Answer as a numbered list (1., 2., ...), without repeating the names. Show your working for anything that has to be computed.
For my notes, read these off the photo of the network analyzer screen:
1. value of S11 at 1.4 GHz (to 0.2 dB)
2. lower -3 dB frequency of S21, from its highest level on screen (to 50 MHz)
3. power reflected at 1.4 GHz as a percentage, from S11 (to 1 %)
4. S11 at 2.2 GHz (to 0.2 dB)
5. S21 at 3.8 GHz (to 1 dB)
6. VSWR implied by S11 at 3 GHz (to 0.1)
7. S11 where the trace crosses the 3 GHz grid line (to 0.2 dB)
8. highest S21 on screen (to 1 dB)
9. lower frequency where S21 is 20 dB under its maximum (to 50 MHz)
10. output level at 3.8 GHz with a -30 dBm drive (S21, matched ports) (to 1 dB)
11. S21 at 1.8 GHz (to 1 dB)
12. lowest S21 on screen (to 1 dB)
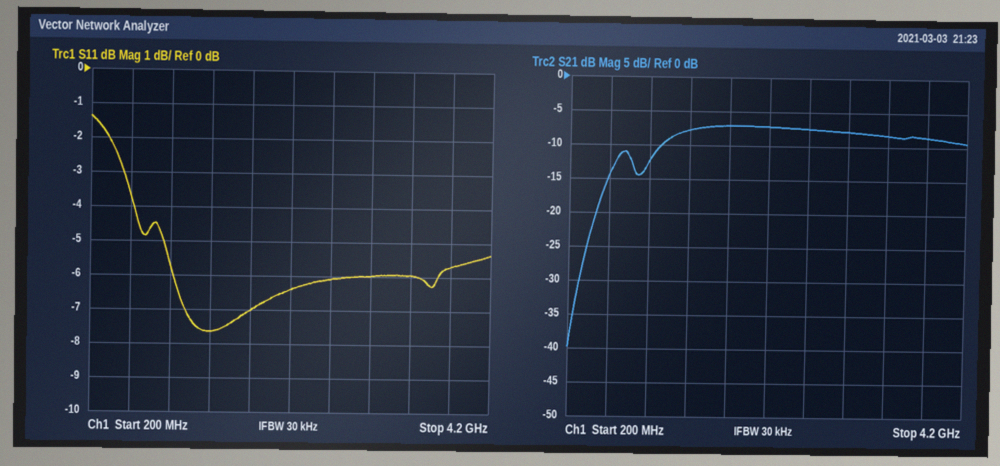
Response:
1. -7.6 dB
2. 1.10 GHz
3. 10^(-7.6/10) ≈ 17 %
4. -6.4 dB
5. -9 dB
6. |Γ| = 10^(-6/20) = 0.5012; VSWR = (1 + 0.5012)/(1 − 0.5012) ≈ 3.0
7. -6.0 dB
8. -7 dB
9. 350 MHz
10. -30 dBm + (-9 dB) = -39 dBm
11. -7 dB
12. -40 dB
